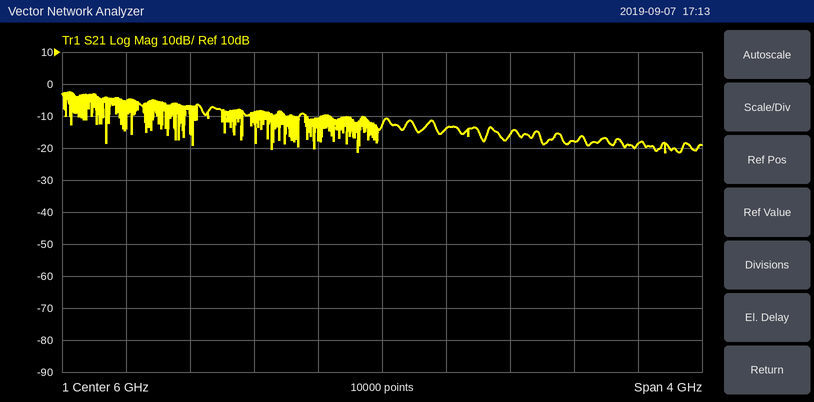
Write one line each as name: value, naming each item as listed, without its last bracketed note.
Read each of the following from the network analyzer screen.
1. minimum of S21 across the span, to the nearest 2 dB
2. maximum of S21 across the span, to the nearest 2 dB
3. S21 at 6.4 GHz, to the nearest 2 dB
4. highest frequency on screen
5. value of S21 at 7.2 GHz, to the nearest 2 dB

minimum of S21 across the span, to the nearest 2 dB: -22 dB
maximum of S21 across the span, to the nearest 2 dB: -2 dB
S21 at 6.4 GHz, to the nearest 2 dB: -14 dB
highest frequency on screen: 8 GHz
value of S21 at 7.2 GHz, to the nearest 2 dB: -18 dB
